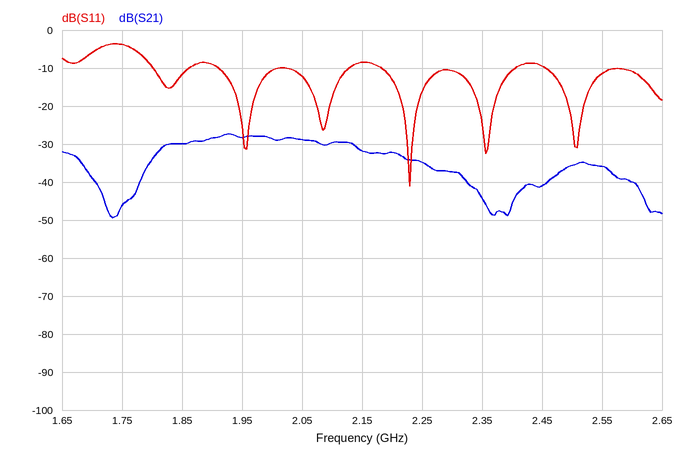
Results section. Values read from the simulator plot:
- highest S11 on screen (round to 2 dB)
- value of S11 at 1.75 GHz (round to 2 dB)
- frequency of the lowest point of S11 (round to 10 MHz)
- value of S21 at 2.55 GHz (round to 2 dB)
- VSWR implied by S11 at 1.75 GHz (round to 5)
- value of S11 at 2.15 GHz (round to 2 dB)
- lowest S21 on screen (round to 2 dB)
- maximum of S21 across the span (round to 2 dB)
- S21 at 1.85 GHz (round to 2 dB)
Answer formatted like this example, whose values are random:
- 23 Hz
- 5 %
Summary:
- -4 dB
- -4 dB
- 2.23 GHz
- -36 dB
- 5
- -8 dB
- -50 dB
- -28 dB
- -30 dB
